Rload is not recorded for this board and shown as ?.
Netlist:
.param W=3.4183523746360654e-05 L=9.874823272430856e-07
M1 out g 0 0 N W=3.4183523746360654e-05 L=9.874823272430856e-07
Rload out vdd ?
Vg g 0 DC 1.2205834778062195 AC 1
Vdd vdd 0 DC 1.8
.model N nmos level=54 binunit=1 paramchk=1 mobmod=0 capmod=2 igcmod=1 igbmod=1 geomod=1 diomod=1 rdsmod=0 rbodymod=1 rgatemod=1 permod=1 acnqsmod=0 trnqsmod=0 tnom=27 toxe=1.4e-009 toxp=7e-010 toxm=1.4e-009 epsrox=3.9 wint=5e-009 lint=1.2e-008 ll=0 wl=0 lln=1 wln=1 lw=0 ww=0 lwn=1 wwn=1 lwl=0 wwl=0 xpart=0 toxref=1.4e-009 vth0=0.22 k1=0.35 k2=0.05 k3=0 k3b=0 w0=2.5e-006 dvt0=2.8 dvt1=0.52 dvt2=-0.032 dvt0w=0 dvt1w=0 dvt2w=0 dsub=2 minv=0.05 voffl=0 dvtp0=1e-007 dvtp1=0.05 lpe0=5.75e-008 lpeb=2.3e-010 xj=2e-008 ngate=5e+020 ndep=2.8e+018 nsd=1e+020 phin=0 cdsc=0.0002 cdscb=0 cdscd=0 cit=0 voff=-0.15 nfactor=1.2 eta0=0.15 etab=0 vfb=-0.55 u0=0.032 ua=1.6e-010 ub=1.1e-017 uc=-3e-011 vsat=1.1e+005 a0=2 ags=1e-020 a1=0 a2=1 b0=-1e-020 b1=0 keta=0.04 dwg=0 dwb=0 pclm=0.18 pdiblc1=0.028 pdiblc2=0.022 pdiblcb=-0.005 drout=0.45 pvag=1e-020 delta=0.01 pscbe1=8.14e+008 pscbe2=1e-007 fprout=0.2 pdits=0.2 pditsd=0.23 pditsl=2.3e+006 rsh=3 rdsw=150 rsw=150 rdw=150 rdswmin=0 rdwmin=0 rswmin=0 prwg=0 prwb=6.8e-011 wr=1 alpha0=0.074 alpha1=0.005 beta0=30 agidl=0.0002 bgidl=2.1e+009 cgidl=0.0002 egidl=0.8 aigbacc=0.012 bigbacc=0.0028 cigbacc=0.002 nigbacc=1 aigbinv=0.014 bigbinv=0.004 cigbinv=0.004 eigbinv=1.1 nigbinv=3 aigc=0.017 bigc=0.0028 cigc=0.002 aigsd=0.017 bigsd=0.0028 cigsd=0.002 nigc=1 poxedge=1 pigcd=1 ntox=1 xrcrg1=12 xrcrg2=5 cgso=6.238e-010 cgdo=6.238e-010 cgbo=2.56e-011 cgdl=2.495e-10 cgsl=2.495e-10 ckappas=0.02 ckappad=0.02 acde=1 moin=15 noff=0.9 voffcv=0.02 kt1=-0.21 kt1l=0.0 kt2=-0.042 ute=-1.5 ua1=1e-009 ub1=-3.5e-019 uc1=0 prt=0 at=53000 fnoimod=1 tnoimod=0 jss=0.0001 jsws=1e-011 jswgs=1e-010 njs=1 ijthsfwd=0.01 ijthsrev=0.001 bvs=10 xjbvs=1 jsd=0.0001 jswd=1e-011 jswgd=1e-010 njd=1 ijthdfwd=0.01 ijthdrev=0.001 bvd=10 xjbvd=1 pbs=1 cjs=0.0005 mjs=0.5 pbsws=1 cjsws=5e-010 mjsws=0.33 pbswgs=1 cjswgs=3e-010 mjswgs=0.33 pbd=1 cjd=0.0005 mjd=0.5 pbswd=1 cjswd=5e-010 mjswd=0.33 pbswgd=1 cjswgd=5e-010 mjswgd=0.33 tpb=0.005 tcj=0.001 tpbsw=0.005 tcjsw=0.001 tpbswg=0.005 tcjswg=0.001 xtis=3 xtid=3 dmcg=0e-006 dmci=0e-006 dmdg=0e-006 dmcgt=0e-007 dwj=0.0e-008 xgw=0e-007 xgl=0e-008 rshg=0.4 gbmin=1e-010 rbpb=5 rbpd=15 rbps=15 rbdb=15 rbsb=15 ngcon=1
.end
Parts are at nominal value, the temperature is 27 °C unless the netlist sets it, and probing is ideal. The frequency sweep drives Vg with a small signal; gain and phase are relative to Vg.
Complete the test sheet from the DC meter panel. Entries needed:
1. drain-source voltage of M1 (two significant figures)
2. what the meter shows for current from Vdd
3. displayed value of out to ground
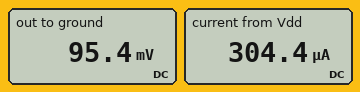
95 mV
304.4 µA
95.4 mV
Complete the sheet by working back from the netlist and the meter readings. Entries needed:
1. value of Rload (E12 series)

5.6 kΩ
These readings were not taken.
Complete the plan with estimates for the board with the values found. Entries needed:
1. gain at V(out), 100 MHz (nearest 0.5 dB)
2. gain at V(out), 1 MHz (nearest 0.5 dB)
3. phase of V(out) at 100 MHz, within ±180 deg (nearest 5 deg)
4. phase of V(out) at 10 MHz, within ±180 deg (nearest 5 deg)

-17.5 dB
-39.5 dB
75 deg
50 deg
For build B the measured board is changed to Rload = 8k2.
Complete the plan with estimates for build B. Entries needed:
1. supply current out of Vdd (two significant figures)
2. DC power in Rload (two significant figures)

210 µA
370 µW
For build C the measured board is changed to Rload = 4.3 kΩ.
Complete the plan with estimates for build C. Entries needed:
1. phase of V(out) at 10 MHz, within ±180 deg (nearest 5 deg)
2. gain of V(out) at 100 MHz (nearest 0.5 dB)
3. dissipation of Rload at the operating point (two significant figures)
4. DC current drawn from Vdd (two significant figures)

55 deg
-17.0 dB
650 µW
390 µA
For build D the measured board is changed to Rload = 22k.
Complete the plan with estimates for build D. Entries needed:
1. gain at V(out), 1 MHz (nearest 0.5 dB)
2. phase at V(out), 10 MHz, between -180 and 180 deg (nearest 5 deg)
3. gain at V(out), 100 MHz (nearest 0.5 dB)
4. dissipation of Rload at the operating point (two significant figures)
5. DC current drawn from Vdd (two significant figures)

-41.5 dB
55 deg
-18.0 dB
140 µW
81 µA
